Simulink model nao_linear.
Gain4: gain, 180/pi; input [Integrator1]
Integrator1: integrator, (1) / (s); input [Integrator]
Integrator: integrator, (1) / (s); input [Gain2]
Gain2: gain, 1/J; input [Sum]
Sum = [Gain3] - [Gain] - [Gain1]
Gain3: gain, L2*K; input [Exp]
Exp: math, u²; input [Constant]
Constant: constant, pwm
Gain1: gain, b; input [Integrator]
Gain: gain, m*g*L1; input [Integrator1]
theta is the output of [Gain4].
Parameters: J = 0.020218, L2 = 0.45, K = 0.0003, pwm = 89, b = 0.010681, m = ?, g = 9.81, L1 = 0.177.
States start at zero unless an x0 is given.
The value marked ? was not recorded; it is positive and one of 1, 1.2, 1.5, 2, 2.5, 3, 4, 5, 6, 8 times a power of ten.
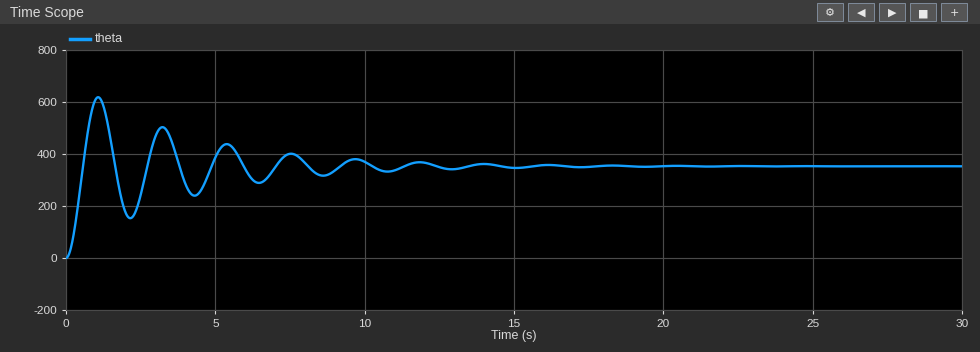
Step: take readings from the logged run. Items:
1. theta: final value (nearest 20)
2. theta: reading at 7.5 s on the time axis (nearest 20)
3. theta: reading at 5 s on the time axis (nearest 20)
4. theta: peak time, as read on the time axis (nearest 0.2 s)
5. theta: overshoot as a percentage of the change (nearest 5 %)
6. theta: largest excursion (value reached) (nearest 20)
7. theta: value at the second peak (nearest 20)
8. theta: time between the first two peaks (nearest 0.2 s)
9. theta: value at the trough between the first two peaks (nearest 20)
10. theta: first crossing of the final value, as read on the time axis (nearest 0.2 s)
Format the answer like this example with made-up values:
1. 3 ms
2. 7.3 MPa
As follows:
1. 360
2. 400
3. 380
4. 1.0 s
5. 75 %
6. 620
7. 500
8. 2.2 s
9. 160
10. 0.6 s
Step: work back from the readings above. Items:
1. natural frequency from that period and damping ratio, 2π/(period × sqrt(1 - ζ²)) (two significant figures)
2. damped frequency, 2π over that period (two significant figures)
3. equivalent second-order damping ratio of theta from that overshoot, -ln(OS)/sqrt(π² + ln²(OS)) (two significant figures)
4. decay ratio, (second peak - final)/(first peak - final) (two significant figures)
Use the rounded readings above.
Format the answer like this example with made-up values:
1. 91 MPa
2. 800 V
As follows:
1. 2.9 rad/s
2. 2.9 rad/s
3. 0.091
4. 0.54
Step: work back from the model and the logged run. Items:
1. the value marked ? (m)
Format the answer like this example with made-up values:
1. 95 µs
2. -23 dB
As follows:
1. 0.1
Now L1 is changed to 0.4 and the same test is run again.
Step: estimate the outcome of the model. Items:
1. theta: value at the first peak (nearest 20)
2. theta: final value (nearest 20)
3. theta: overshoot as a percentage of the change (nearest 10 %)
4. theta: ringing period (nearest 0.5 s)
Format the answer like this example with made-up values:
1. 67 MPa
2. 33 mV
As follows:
1. 280
2. 160
3. 80 %
4. 1.5 s
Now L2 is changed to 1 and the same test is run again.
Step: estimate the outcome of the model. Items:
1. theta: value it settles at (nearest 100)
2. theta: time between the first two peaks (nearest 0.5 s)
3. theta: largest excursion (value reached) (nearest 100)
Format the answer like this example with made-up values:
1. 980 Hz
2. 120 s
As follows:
1. 800
2. 2.0 s
3. 1400
